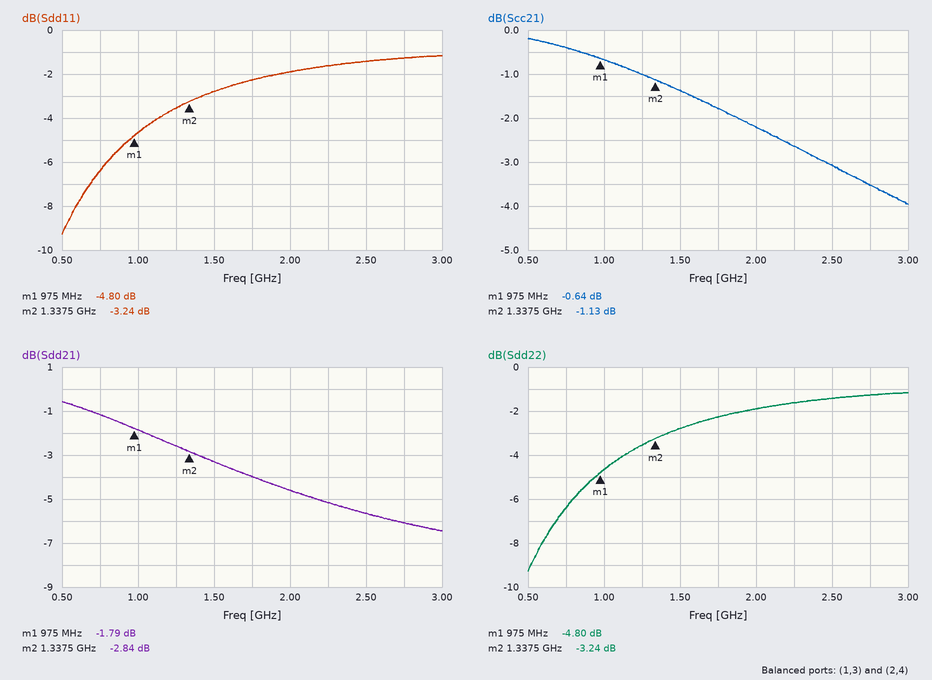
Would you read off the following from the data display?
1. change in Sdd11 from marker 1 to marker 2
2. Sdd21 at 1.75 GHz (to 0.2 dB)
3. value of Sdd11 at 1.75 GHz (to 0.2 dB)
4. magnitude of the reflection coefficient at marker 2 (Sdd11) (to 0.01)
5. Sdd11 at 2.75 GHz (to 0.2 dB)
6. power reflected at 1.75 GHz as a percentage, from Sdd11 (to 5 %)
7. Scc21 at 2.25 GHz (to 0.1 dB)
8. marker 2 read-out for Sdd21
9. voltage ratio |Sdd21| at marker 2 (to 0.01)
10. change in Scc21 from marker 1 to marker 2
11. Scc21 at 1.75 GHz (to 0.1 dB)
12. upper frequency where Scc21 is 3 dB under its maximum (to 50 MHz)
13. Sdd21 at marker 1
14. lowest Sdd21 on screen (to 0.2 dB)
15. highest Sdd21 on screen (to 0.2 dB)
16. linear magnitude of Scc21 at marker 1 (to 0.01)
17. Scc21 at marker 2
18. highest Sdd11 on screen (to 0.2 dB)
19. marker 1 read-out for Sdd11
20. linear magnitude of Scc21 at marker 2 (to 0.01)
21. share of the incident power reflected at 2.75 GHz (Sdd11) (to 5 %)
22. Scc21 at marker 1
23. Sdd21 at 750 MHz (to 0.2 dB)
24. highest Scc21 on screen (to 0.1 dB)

1.56 dB
-4.0 dB
-2.2 dB
0.69
-1.2 dB
60 %
-2.6 dB
-2.84 dB
0.72
-0.49 dB
-1.8 dB
2.55 GHz
-1.79 dB
-6.4 dB
-0.6 dB
0.93
-1.13 dB
-1.2 dB
-4.80 dB
0.88
75 %
-0.64 dB
-1.2 dB
-0.2 dB
